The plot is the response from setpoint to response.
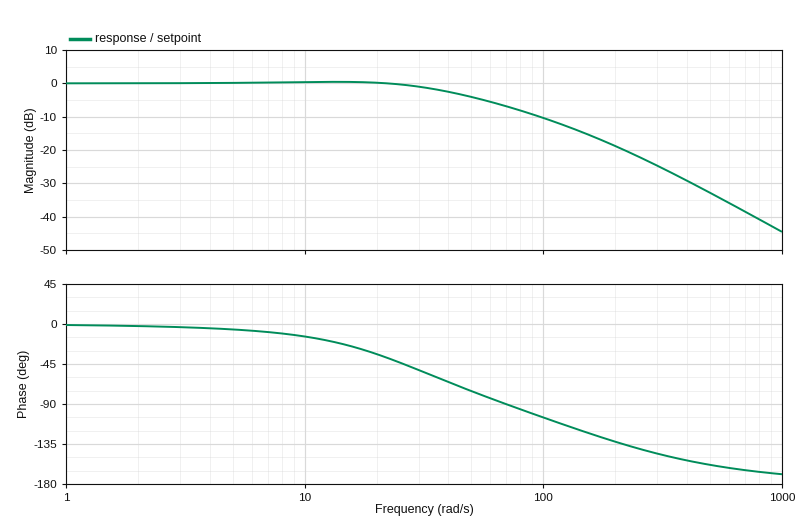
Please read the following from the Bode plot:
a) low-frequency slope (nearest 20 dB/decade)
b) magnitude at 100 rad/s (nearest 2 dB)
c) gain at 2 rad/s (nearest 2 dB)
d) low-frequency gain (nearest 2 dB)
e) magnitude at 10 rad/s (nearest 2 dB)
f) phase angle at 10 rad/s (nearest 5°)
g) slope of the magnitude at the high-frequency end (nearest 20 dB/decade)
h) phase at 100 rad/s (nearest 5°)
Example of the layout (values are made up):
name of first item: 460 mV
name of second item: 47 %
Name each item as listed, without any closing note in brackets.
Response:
low-frequency slope: 0 dB/decade
magnitude at 100 rad/s: -10 dB
gain at 2 rad/s: 0 dB
low-frequency gain: 0 dB
magnitude at 10 rad/s: 0 dB
phase angle at 10 rad/s: -15°
slope of the magnitude at the high-frequency end: -40 dB/decade
phase at 100 rad/s: -105°
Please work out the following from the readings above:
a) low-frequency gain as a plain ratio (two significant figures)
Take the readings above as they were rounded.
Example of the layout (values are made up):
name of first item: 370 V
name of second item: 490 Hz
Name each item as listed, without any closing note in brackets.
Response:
low-frequency gain as a plain ratio: 1.0
